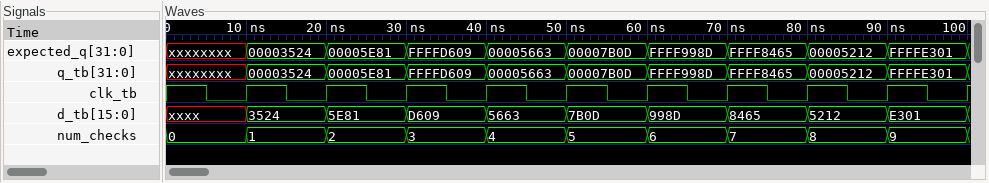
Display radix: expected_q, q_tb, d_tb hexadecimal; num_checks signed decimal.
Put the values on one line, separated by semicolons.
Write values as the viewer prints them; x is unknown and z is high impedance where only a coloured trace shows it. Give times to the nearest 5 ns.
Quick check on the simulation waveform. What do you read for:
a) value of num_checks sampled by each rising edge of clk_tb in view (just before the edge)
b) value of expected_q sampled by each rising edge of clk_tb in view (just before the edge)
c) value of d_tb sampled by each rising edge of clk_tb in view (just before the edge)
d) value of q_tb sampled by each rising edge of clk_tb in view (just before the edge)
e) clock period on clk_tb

0, 1, 2, 3, 4, 5, 6, 7, 8, 9; xxxxxxxx, 00003524, 00005E81, FFFFD609, 00005663, 00007B0D, FFFF998D, FFFF8465, 00005212, FFFFE301; xxxx, 3524, 5E81, D609, 5663, 7B0D, 998D, 8465, 5212, E301; xxxxxxxx, 00003524, 00005E81, FFFFD609, 00005663, 00007B0D, FFFF998D, FFFF8465, 00005212, FFFFE301; 10 ns
